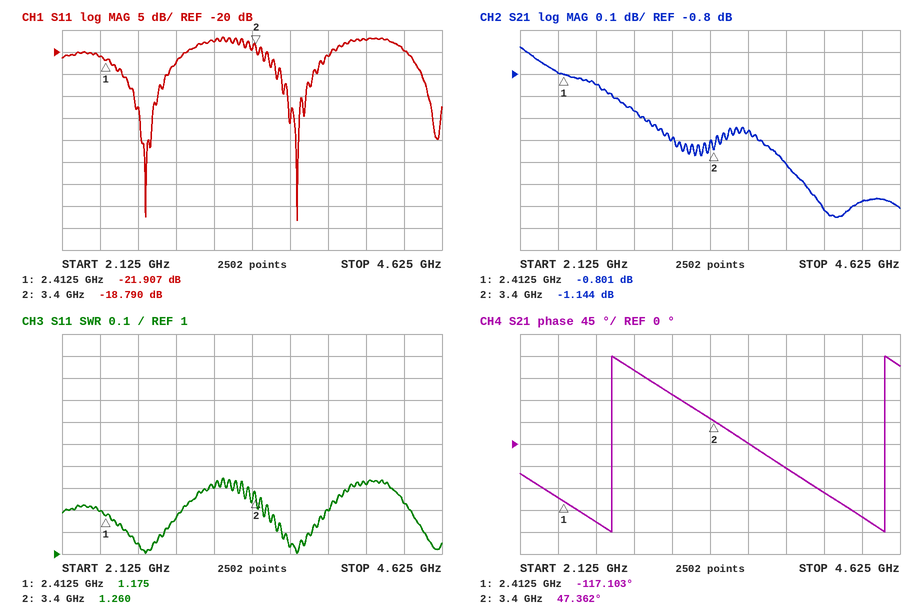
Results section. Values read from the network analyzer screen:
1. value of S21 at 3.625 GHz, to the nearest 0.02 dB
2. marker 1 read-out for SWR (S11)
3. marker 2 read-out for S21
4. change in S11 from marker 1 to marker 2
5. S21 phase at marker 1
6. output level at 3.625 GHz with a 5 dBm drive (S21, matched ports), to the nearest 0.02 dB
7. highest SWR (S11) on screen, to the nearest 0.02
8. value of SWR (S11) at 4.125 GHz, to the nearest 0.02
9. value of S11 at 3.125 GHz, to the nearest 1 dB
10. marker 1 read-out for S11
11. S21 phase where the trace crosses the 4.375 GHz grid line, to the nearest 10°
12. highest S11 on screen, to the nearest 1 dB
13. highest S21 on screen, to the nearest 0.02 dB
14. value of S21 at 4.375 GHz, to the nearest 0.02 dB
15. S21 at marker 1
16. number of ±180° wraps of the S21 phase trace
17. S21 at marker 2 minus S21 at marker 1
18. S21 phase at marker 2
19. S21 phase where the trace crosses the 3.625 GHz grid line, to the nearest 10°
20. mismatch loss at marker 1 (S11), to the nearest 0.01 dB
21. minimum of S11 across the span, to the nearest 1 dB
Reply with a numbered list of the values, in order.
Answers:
1. -1.06 dB
2. 1.175
3. -1.144 dB
4. 3.117 dB
5. -117.103°
6. 3.94 dBm
7. 1.34
8. 1.32
9. -18 dB
10. -21.907 dB
11. -150°
12. -17 dB
13. -0.68 dB
14. -1.38 dB
15. -0.801 dB
16. 2
17. -0.343 dB
18. 47.362°
19. 0°
20. 0.03 dB
21. -58 dB
